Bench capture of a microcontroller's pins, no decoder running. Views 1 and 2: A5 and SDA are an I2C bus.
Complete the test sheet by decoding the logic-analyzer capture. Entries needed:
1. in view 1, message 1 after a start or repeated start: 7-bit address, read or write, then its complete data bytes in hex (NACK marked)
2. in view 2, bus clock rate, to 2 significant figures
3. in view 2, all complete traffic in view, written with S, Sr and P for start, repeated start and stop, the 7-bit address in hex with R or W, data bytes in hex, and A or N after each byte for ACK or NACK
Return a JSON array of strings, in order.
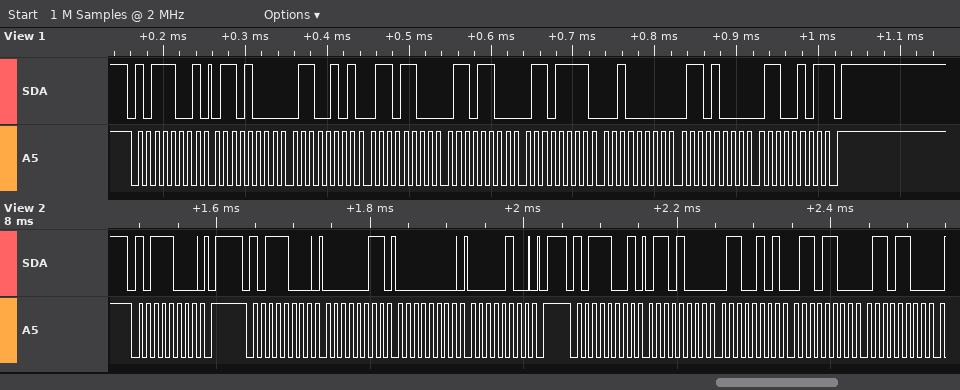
["0x5C read: 68 65 6C 6C 6F 20 68 65 NACK", "100 kHz", "S 5CW A P S 5CW A 03 A 00 A 04 A P S 5CR A 68 A 65 A 6C A 6C A"]
